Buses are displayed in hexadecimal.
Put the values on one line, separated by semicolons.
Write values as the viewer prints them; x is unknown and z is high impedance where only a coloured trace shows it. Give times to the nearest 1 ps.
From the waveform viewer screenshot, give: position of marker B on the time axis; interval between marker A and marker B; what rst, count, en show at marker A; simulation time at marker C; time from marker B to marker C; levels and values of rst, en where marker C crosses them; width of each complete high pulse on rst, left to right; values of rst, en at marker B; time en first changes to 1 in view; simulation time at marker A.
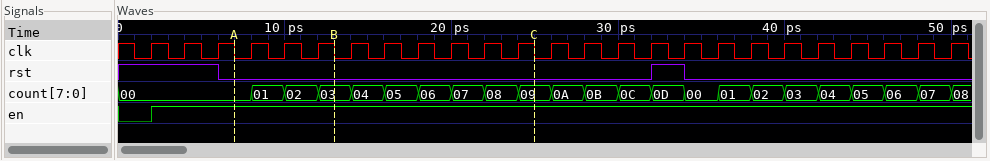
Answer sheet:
13 ps; 6 ps; rst=0, count=00, en=1; 25 ps; 12 ps; rst=0, en=1; 2 ps; rst=0, en=1; 2 ps; 7 ps
